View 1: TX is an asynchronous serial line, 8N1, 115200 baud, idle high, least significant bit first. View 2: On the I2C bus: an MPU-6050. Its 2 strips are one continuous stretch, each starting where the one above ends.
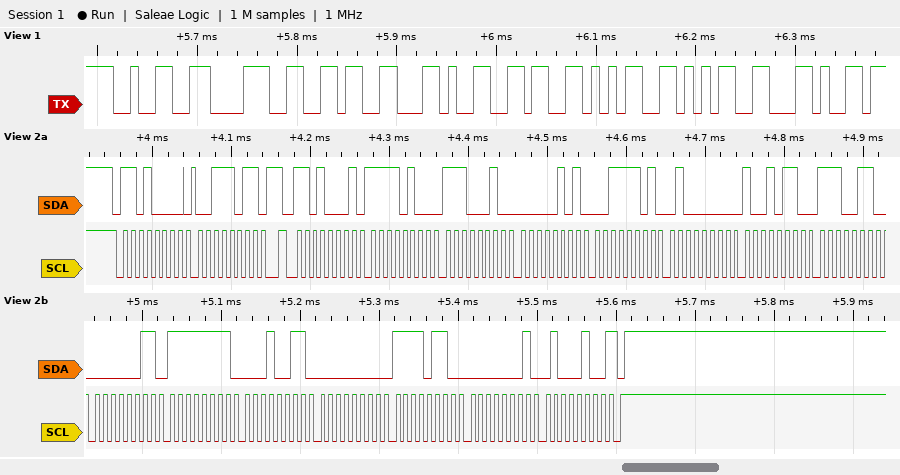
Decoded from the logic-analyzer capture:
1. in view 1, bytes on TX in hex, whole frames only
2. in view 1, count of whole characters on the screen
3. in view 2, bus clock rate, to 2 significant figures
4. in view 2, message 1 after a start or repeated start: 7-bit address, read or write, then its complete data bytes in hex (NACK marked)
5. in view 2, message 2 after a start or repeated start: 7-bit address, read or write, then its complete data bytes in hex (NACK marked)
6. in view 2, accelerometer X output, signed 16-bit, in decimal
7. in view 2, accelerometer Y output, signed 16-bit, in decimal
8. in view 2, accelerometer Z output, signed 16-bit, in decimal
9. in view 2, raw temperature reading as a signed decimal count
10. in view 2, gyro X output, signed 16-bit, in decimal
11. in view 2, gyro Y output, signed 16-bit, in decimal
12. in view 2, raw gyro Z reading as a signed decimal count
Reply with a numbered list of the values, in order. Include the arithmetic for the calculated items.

1. 32 38 36 2C 36 35 35 2C
2. 8
3. 100 kHz
4. 0x68 write: 3B
5. 0x68 read: F4 E2 05 3D 40 96 E6 03 FF 13 00 F6 01 44 NACK
6. 0xF4E2 = -2846
7. 0x053D = 1341
8. 0x4096 = 16534
9. 0xE603 = -6653
10. 0xFF13 = -237
11. 0x00F6 = 246
12. 0x0144 = 324
